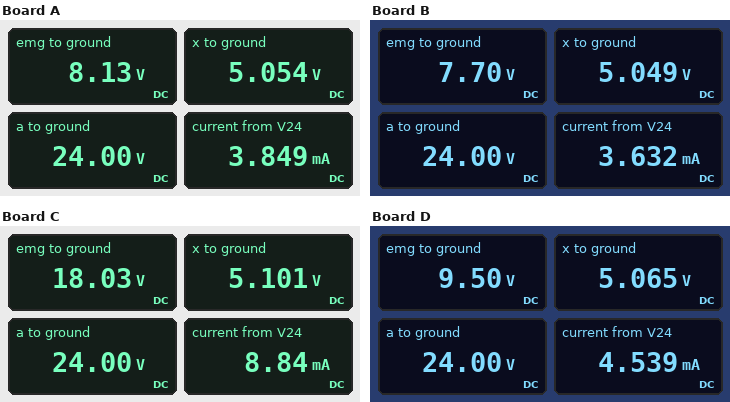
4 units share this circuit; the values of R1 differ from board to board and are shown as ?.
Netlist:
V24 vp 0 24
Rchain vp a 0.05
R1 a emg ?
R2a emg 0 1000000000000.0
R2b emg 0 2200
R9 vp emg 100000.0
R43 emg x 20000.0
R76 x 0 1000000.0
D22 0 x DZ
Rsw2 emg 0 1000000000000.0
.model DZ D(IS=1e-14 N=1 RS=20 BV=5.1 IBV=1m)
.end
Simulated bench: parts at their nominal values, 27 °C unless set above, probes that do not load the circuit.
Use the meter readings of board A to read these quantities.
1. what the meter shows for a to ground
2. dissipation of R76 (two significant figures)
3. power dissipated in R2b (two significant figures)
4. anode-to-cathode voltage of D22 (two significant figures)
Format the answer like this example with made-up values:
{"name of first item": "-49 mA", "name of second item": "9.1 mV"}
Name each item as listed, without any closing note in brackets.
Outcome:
{"what the meter shows for a to ground": "24.00 V", "dissipation of R76": "26 µW", "power dissipated in R2b": "30 mW", "anode-to-cathode voltage of D22": "-5.1 V"}
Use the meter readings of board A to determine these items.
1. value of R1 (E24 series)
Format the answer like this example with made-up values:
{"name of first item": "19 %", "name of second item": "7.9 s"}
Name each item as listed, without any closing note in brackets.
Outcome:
{"value of R1": "4.3 kΩ"}
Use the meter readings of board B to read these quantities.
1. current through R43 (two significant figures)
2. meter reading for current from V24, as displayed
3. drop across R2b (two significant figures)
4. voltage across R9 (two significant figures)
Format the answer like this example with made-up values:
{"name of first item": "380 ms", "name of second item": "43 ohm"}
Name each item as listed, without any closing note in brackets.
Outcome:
{"current through R43": "130 µA", "meter reading for current from V24, as displayed": "3.632 mA", "drop across R2b": "7.7 V", "voltage across R9": "16 V"}
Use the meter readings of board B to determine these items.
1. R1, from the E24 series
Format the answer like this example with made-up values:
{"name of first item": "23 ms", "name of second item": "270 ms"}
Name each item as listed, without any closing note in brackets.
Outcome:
{"R1, from the E24 series": "4.7 kΩ"}
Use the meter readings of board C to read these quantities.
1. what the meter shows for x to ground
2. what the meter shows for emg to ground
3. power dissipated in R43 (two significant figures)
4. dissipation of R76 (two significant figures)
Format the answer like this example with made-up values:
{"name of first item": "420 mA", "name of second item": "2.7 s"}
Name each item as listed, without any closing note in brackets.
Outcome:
{"what the meter shows for x to ground": "5.101 V", "what the meter shows for emg to ground": "18.03 V", "power dissipated in R43": "8.4 mW", "dissipation of R76": "26 µW"}
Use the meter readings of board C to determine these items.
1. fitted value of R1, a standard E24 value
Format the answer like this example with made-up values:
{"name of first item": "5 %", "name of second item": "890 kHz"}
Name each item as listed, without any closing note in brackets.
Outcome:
{"fitted value of R1, a standard E24 value": "680 Ω"}
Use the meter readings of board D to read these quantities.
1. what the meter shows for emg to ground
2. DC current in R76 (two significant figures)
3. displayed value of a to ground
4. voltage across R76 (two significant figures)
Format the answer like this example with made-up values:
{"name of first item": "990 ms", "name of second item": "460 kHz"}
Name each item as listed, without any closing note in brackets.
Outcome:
{"what the meter shows for emg to ground": "9.50 V", "DC current in R76": "5.1 µA", "displayed value of a to ground": "24.00 V", "voltage across R76": "5.1 V"}
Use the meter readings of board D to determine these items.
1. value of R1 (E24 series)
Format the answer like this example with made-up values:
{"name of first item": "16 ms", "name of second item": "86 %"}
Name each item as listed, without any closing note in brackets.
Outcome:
{"value of R1": "3.3 kΩ"}
